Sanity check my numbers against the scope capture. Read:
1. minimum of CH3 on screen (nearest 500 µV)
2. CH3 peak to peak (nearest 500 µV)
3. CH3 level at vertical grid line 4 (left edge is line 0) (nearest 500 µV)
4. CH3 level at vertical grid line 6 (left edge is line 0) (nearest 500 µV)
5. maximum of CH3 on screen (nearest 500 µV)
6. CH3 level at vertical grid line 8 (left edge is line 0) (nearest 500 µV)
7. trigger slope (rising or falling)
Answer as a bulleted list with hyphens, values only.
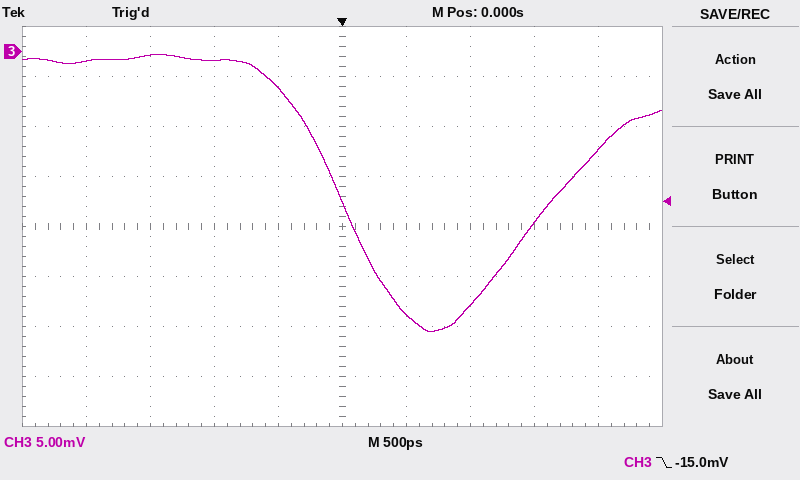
- -28.0 mV
- 27.5 mV
- -3.5 mV
- -26.5 mV
- -500 µV
- -17.0 mV
- falling
